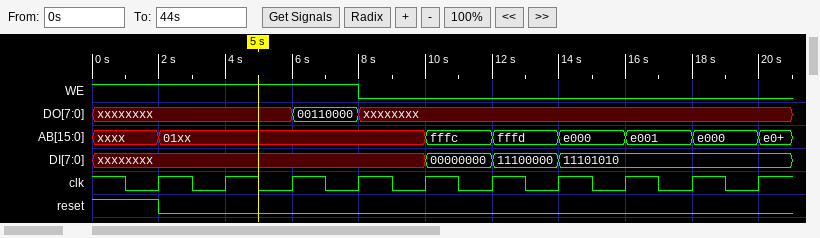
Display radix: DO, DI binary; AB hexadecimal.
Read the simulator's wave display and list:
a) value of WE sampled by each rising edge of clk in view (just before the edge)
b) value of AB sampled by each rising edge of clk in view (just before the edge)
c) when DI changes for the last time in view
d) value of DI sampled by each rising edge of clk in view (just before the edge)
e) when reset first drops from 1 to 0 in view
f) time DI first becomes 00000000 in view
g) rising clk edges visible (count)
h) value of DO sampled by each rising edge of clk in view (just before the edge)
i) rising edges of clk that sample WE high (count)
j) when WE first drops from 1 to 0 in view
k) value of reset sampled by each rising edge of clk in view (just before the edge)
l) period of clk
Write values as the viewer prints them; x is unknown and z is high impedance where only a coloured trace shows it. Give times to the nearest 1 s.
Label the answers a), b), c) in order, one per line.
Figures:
a) 1 1 1 1 0 0 0 0 0 0
b) xxxx, 01xx, 01xx, 01xx, 01xx, fffc, fffd, e000, e001, e000
c) 14 s
d) xxxxxxxx, xxxxxxxx, xxxxxxxx, xxxxxxxx, xxxxxxxx, 00000000, 11100000, 11101010, 11101010, 11101010
e) 2 s
f) 10 s
g) 10
h) xxxxxxxx, xxxxxxxx, xxxxxxxx, 00110000, xxxxxxxx, xxxxxxxx, xxxxxxxx, xxxxxxxx, xxxxxxxx, xxxxxxxx
i) 4
j) 8 s
k) 1 0 0 0 0 0 0 0 0 0
l) 2 s
